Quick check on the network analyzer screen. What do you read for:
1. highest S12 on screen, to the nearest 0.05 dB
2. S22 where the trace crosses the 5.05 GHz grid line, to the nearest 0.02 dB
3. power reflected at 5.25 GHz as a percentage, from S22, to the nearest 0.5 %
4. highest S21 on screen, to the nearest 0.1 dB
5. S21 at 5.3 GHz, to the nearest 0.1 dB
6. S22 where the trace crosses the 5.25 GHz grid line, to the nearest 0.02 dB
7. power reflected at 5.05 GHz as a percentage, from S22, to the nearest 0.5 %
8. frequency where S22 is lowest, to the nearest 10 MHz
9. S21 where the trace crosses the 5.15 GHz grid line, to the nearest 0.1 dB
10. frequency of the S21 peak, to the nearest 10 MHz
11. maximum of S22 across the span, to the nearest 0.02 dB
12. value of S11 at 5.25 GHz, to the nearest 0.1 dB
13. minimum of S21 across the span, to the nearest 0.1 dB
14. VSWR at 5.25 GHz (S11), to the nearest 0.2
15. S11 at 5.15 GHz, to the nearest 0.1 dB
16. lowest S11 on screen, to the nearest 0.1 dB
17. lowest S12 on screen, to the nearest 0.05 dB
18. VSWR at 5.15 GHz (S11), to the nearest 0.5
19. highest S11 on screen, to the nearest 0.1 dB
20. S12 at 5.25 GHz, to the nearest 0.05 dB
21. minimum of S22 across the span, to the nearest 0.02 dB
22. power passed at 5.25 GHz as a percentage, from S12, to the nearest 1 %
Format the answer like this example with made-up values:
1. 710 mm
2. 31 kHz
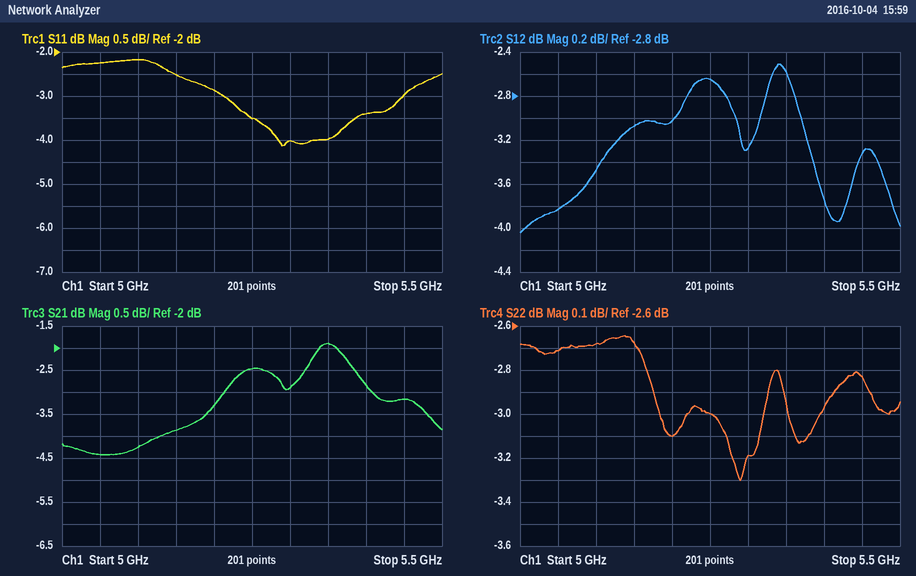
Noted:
1. -2.50 dB
2. -2.72 dB
3. 50.0 %
4. -1.9 dB
5. -2.9 dB
6. -3.00 dB
7. 53.5 %
8. 5.29 GHz
9. -3.9 dB
10. 5.35 GHz
11. -2.64 dB
12. -3.5 dB
13. -4.4 dB
14. 5.0
15. -2.5 dB
16. -4.1 dB
17. -4.05 dB
18. 7.0
19. -2.2 dB
20. -2.65 dB
21. -3.30 dB
22. 54 %
